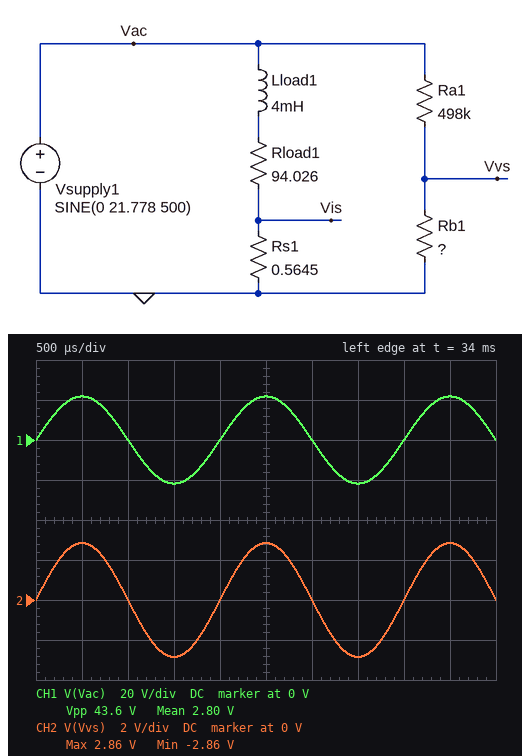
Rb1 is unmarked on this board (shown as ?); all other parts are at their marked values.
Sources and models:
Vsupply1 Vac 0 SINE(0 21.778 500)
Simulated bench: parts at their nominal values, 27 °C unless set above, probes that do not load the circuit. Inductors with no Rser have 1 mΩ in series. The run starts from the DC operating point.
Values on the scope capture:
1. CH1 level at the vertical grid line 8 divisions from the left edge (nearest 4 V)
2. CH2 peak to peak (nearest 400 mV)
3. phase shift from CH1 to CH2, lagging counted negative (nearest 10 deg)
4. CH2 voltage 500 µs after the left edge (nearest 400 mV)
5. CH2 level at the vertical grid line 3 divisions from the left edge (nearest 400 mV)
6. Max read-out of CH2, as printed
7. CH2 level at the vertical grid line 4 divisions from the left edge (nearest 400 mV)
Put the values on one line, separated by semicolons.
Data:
0 V; 5.6 V; 0 deg; 2.8 V; -2.8 V; 2.86 V; 0 V
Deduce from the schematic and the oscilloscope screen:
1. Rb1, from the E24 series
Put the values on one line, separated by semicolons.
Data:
75 kΩ
